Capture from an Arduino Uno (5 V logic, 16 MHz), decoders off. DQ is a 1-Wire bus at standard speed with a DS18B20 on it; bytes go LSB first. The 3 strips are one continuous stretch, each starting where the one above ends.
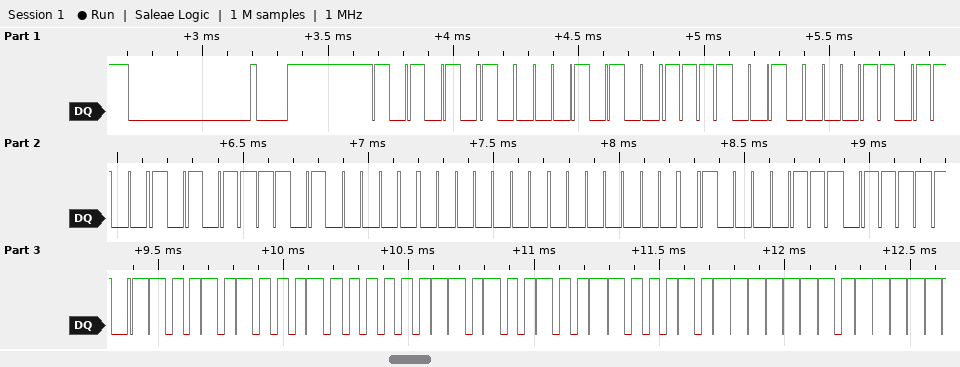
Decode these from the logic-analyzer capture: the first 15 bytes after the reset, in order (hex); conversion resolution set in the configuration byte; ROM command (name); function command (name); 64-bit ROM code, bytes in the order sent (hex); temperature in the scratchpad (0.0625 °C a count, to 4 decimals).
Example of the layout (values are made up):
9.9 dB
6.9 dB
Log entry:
55 28 4F D8 D4 0B 00 00 E1 BE 29 02 4B 46 7F
12 bits
Match ROM
Read Scratchpad
28 4F D8 D4 0B 00 00 E1
34.5625 °C
